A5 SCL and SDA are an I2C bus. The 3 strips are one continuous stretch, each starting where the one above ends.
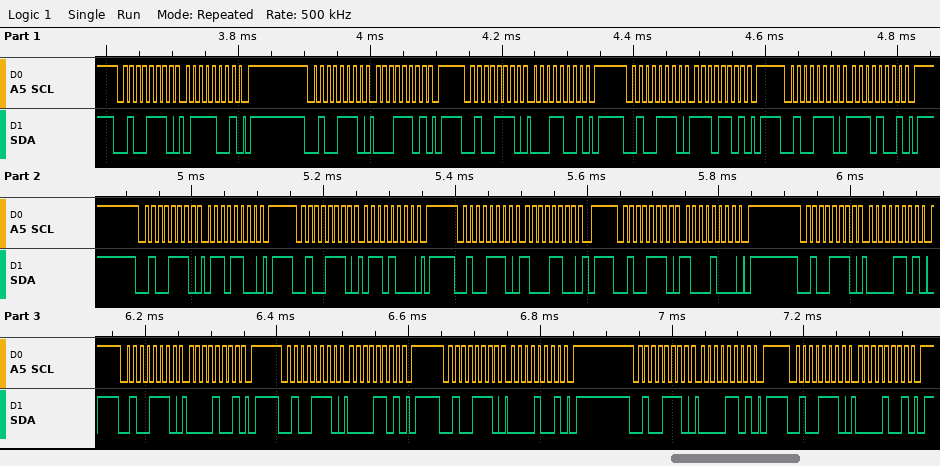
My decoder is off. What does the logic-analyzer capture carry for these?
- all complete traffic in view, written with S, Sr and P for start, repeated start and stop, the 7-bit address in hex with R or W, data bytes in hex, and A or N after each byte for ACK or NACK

S 27W A 79 A P S 27W A 1D A P S 27W A 19 A P S 27W A ED A P S 27W A E9 A P S 27W A 6C A P S 27W A 68 A P S 27W A 8C A P S 27W A 88 A P S 27W A 0D A P S 27W A 09 A P S 27W A 0D A P S 27W A 09 A P S 27W A 0D A P S 27W A 09 A P
